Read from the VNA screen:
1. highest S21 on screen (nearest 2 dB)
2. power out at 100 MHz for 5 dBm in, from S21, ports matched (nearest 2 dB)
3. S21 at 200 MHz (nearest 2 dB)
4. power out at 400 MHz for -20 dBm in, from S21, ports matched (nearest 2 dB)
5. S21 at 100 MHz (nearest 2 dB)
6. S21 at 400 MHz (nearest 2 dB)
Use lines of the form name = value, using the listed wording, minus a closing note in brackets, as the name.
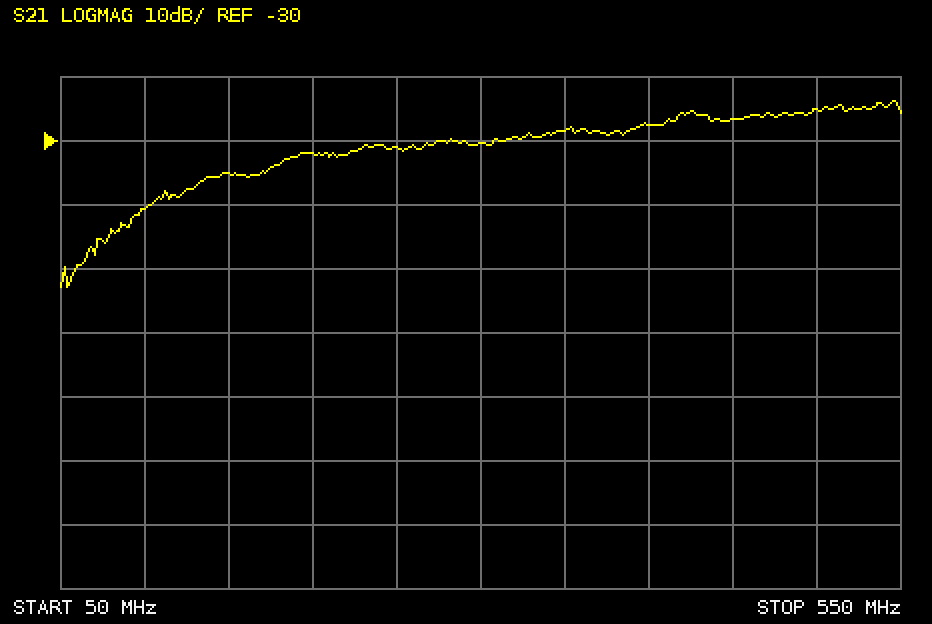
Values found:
highest S21 on screen = -24 dB
power out at 100 MHz for 5 dBm in, from S21, ports matched = -36 dBm
S21 at 200 MHz = -32 dB
power out at 400 MHz for -20 dBm in, from S21, ports matched = -48 dBm
S21 at 100 MHz = -40 dB
S21 at 400 MHz = -28 dB
